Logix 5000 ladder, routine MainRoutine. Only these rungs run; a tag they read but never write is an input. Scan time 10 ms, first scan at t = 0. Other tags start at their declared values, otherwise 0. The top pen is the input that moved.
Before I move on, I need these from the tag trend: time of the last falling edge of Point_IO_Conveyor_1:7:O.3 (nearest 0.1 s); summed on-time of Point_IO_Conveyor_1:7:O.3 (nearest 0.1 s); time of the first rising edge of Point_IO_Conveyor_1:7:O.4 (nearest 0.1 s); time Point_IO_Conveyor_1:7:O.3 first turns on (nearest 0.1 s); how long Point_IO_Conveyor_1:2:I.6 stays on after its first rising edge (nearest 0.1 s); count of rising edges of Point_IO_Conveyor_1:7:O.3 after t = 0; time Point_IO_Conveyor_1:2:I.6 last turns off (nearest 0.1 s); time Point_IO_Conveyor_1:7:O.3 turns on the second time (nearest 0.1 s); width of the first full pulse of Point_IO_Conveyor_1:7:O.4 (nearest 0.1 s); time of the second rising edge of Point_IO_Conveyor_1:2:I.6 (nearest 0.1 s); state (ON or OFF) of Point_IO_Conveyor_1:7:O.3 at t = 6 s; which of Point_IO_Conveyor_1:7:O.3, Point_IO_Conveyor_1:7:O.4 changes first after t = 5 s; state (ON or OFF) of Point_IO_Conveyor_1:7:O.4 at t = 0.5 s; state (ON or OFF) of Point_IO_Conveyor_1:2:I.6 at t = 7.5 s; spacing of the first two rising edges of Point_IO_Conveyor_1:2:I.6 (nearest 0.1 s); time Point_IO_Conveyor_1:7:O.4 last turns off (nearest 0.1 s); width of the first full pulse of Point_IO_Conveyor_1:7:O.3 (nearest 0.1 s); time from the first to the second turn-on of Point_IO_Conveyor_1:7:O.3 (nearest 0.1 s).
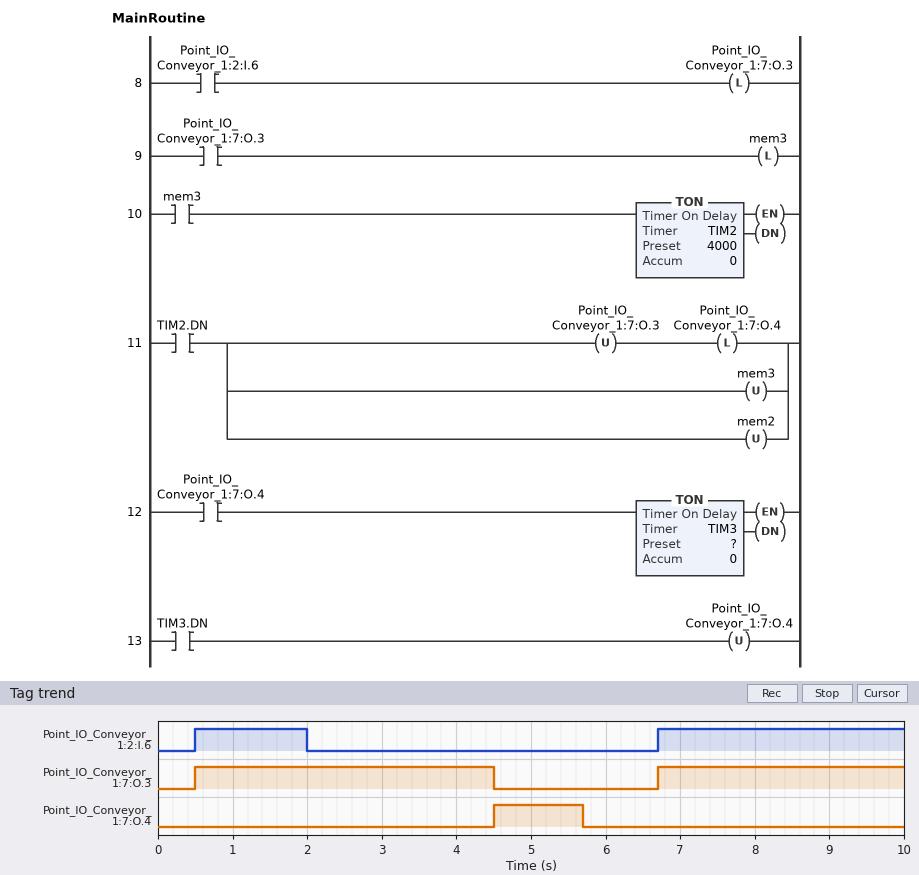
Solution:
4.5 s
7.3 s
4.5 s
0.5 s
1.5 s
2
2.0 s
6.7 s
1.2 s
6.7 s
OFF
Point_IO_Conveyor_1:7:O.4
OFF
ON
6.2 s
5.7 s
4.0 s
6.2 s
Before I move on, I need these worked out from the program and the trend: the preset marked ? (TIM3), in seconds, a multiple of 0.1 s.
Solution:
1.2 s
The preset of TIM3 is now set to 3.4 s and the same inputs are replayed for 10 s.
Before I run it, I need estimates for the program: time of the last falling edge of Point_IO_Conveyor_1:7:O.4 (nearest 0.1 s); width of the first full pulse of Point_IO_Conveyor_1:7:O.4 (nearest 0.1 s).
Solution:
7.9 s
3.4 s
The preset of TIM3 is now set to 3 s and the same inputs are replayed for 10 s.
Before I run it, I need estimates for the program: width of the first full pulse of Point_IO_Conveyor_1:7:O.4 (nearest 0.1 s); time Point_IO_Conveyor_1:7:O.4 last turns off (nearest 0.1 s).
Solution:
3.0 s
7.5 s
